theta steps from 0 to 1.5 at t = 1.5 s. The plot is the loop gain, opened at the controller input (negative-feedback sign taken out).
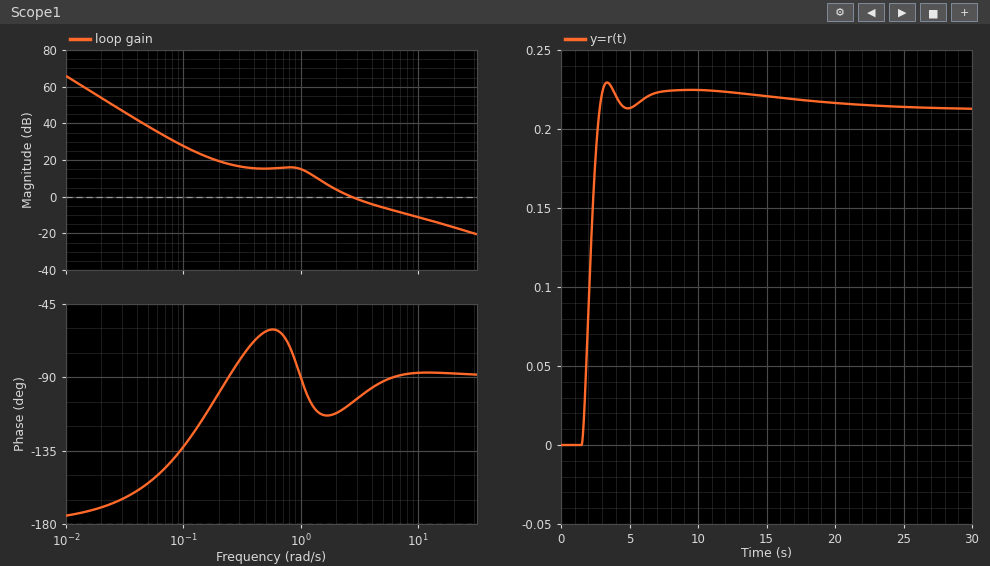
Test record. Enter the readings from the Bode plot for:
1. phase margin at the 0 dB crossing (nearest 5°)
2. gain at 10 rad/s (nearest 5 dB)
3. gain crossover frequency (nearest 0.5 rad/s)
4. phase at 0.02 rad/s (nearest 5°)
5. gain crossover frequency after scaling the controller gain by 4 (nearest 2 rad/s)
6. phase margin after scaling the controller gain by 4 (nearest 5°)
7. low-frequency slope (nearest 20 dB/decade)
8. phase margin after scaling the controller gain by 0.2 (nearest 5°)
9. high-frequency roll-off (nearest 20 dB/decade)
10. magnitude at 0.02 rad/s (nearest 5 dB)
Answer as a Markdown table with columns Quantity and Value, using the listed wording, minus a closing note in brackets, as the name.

| Quantity | Value |
|---|---|
| phase margin at the 0 dB crossing | 75° |
| gain at 10 rad/s | -10 dB |
| gain crossover frequency | 2.5 rad/s |
| phase at 0.02 rad/s | -170° |
| gain crossover frequency after scaling the controller gain by 4 | 12 rad/s |
| phase margin after scaling the controller gain by 4 | 95° |
| low-frequency slope | -40 dB/decade |
| phase margin after scaling the controller gain by 0.2 | 80° |
| high-frequency roll-off | -20 dB/decade |
| magnitude at 0.02 rad/s | 55 dB |
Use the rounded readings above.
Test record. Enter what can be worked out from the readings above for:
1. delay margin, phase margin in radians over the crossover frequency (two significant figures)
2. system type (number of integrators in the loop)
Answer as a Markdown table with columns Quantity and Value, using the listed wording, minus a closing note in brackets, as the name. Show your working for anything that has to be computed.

| Quantity | Value |
|---|---|
| delay margin, phase margin in radians over the crossover frequency | 75 × π / 180 / 2.5 = 0.52 s |
| system type | 2 |
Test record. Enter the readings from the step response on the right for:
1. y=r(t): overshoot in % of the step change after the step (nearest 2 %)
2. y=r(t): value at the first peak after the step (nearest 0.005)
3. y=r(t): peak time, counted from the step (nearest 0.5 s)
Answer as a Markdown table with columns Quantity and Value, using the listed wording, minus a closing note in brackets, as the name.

| Quantity | Value |
|---|---|
| y=r(t): overshoot in % of the step change after the step | 8 % |
| y=r(t): value at the first peak after the step | 0.230 |
| y=r(t): peak time, counted from the step | 2.0 s |
